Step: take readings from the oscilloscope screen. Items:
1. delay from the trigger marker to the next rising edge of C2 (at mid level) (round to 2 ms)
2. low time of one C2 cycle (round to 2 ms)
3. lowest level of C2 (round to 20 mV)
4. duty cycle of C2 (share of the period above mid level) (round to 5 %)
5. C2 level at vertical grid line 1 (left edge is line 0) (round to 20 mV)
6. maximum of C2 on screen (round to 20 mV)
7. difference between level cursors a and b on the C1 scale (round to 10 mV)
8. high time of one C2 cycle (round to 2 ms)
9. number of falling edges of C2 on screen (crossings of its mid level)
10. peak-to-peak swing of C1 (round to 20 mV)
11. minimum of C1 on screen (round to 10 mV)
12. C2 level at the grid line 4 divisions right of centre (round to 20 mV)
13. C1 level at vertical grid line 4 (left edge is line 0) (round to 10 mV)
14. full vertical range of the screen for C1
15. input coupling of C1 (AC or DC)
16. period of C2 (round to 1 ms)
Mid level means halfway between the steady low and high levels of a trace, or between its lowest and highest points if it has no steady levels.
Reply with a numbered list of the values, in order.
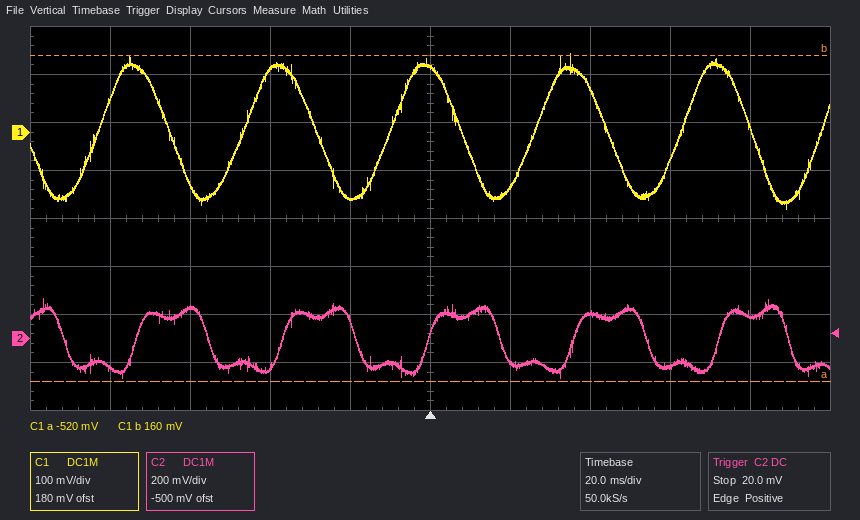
1. 36 ms
2. 18 ms
3. -160 mV
4. 50 %
5. -120 mV
6. 160 mV
7. 680 mV
8. 18 ms
9. 6
10. 320 mV
11. -160 mV
12. 100 mV
13. -140 mV
14. 800 mV
15. DC
16. 36 ms
